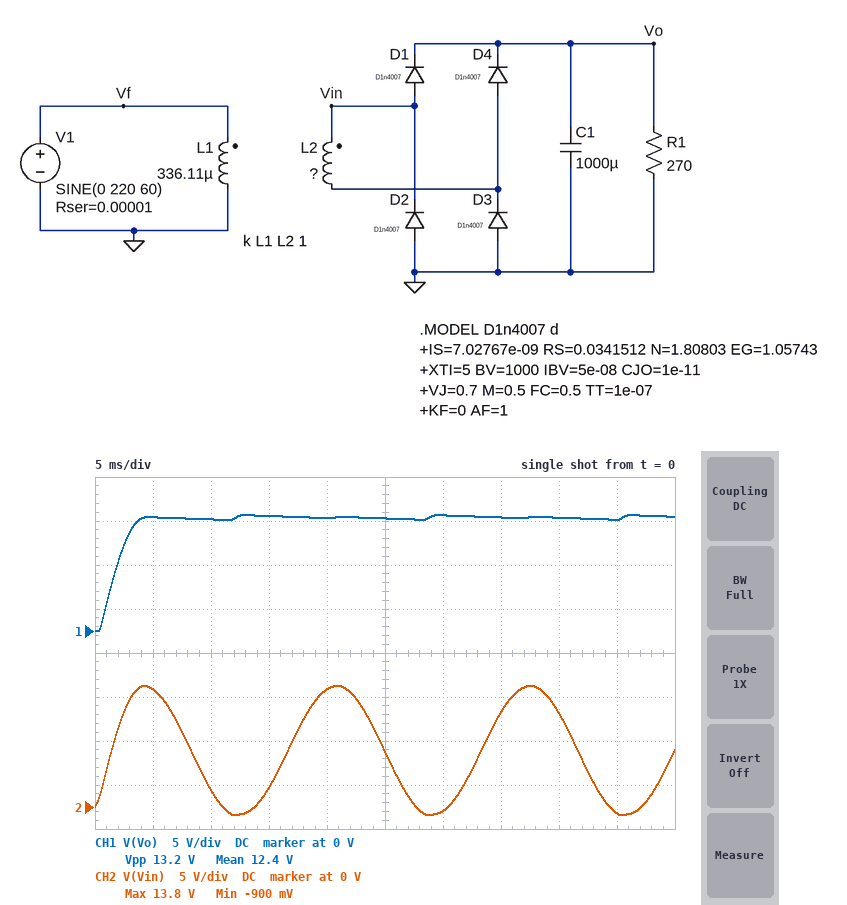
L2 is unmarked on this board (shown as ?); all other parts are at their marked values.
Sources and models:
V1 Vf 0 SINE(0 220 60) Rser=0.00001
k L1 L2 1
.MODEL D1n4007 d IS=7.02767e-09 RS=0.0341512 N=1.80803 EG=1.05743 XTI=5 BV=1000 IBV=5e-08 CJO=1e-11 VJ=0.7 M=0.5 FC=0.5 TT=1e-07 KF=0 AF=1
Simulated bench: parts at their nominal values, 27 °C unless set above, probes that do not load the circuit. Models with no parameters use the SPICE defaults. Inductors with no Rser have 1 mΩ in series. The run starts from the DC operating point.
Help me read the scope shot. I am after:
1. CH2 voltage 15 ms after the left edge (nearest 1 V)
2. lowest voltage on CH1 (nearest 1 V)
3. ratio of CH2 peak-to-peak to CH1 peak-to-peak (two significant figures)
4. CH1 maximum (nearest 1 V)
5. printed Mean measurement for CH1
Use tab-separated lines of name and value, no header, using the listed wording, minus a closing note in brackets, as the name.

CH2 voltage 15 ms after the left edge	2 V
lowest voltage on CH1	0 V
ratio of CH2 peak-to-peak to CH1 peak-to-peak	1.1
CH1 maximum	13 V
printed Mean measurement for CH1	12.4 V
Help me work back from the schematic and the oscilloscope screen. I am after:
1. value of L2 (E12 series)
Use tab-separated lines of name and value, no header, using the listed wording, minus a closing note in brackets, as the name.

value of L2	1.5 µH
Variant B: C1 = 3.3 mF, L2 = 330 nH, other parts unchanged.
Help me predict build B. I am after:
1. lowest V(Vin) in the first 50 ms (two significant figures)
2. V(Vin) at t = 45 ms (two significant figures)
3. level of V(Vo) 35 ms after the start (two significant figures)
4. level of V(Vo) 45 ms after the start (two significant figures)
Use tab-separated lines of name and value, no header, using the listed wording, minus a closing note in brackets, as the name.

lowest V(Vin) in the first 50 ms	-890 mV
V(Vin) at t = 45 ms	-690 mV
level of V(Vo) 35 ms after the start	5.3 V
level of V(Vo) 45 ms after the start	5.2 V
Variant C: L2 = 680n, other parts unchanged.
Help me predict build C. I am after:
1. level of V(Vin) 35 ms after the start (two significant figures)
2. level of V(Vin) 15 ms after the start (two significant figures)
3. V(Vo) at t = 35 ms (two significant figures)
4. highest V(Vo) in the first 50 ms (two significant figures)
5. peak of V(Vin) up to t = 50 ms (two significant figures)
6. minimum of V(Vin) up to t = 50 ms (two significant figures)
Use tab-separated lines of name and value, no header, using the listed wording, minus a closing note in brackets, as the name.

level of V(Vin) 35 ms after the start	7.0 V
level of V(Vin) 15 ms after the start	1.2 V
V(Vo) at t = 35 ms	8.2 V
highest V(Vo) in the first 50 ms	8.4 V
peak of V(Vin) up to t = 50 ms	9.0 V
minimum of V(Vin) up to t = 50 ms	-870 mV
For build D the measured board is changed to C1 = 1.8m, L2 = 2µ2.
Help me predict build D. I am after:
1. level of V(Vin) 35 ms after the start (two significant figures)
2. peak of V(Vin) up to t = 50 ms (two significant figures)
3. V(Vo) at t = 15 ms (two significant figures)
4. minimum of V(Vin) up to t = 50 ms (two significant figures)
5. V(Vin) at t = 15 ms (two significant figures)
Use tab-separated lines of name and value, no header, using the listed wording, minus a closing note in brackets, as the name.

level of V(Vin) 35 ms after the start	13 V
peak of V(Vin) up to t = 50 ms	17 V
V(Vo) at t = 15 ms	16 V
minimum of V(Vin) up to t = 50 ms	-950 mV
V(Vin) at t = 15 ms	2.8 V
